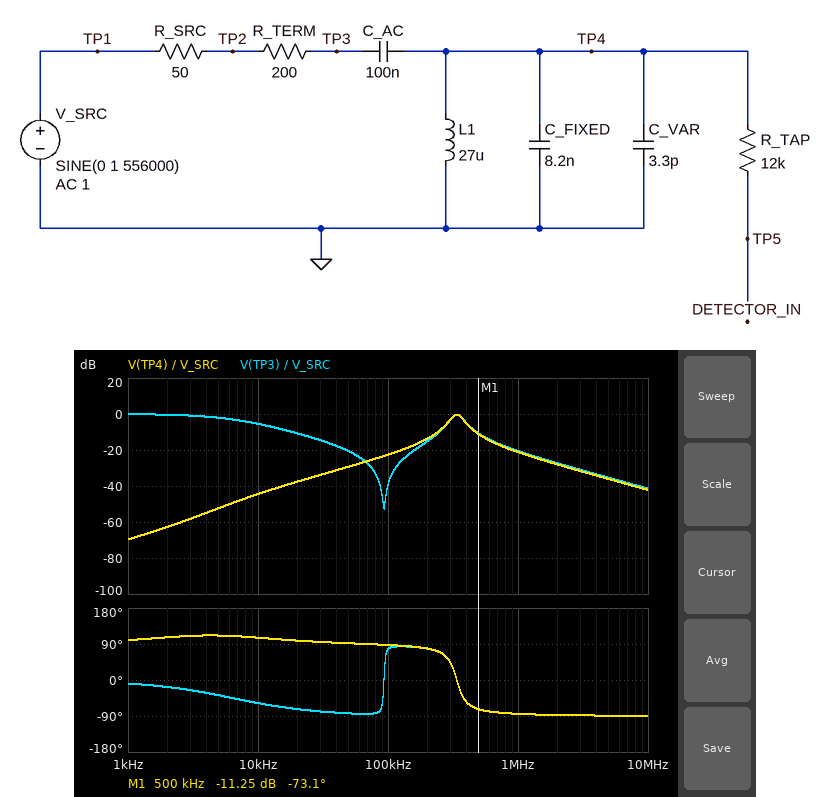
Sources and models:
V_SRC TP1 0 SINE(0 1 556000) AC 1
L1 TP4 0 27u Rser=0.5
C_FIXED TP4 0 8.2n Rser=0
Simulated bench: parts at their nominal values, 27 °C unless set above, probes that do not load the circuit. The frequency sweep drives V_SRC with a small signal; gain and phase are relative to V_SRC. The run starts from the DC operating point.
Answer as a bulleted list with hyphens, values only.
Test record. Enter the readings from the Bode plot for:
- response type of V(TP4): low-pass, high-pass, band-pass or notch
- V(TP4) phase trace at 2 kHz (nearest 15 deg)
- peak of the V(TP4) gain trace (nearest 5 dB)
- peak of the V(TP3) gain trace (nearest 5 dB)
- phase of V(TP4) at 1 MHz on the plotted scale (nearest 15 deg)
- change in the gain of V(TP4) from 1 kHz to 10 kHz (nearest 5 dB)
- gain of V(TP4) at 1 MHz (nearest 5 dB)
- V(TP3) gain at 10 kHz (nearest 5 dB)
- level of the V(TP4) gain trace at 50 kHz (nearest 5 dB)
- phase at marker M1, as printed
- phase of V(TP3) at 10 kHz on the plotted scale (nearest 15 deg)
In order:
- band-pass
- 105 deg
- 0 dB
- 0 dB
- -90 deg
- 25 dB
- -20 dB
- -5 dB
- -30 dB
- -73.1 deg
- -60 deg
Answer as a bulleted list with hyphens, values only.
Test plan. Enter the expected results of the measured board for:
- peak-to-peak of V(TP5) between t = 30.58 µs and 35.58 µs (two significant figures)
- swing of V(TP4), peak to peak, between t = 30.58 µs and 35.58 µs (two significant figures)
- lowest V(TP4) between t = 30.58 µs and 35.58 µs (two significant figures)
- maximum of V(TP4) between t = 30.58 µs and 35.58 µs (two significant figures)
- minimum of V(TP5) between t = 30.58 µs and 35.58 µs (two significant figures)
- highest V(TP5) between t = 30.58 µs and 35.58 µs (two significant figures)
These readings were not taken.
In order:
- 430 mV
- 430 mV
- -220 mV
- 220 mV
- -220 mV
- 220 mV
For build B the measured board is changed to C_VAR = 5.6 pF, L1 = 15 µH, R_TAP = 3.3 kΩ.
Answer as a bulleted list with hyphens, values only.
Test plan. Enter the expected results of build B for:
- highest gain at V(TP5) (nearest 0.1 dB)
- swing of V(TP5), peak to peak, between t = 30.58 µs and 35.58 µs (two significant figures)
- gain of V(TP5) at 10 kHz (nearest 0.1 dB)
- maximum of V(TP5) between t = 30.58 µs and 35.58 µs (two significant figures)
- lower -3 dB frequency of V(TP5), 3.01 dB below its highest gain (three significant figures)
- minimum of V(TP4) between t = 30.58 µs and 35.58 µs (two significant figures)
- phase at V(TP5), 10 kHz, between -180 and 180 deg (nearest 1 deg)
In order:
- -0.6 dB
- 760 mV
- -48.9 dB
- 380 mV
- 414 kHz
- -380 mV
- 94 deg
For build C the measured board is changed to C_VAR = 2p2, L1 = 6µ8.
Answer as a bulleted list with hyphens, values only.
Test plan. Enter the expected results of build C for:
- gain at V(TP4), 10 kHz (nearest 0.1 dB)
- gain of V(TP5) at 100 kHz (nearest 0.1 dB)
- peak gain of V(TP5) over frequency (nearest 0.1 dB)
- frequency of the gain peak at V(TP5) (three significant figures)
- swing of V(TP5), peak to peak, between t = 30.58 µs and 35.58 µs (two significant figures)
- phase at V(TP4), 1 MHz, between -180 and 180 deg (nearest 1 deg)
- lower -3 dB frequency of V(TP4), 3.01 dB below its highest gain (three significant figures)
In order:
- -53.1 dB
- -35.1 dB
- -1.2 dB
- 674 kHz
- 560 mV
- -81 deg
- 631 kHz
